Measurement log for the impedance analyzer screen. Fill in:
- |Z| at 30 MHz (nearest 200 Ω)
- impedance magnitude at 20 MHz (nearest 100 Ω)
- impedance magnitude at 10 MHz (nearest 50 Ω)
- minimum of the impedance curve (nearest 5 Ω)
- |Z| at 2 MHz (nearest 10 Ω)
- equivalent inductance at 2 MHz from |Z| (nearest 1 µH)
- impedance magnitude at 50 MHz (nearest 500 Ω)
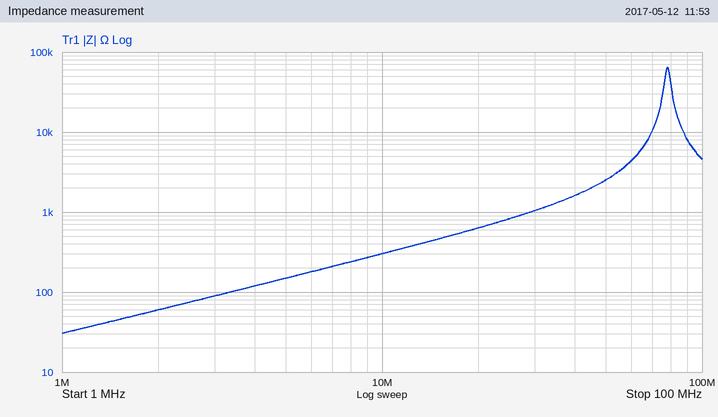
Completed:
1.0 kΩ
600 Ω
300 Ω
30 Ω
60 Ω
5 µH
2.5 kΩ
